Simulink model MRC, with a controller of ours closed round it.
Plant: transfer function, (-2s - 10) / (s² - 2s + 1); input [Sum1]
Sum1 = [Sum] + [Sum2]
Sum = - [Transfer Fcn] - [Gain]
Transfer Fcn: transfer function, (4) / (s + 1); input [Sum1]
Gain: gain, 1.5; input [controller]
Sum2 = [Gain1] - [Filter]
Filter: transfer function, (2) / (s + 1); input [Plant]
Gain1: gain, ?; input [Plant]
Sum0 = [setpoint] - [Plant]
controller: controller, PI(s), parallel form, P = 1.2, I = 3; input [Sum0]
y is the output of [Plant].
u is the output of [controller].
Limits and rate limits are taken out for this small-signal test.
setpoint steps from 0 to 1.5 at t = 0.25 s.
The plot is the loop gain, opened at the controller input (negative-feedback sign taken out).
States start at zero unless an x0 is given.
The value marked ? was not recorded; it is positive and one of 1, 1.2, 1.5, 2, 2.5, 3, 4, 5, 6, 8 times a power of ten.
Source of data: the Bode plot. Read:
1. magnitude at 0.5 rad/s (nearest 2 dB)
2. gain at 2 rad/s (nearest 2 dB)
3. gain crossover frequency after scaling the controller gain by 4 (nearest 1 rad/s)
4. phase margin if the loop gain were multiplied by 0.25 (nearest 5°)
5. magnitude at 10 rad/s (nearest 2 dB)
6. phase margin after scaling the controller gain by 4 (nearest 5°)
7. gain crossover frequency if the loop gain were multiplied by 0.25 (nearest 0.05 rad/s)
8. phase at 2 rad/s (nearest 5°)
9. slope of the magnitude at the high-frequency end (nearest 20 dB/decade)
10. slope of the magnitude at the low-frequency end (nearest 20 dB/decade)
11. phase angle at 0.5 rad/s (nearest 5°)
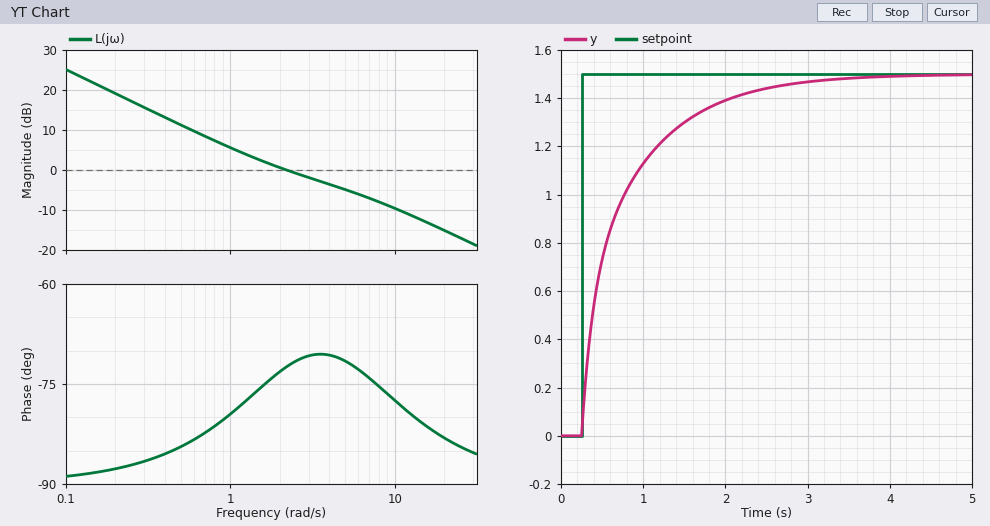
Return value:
12 dB
0 dB
14 rad/s
95°
-10 dB
100°
0.45 rad/s
-75°
-20 dB/decade
-20 dB/decade
-85°
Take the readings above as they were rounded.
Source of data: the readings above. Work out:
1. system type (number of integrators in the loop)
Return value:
1
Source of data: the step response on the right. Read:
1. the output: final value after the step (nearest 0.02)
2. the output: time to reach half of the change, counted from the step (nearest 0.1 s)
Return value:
1.50
0.3 s
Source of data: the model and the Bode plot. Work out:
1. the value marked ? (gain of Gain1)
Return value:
4
